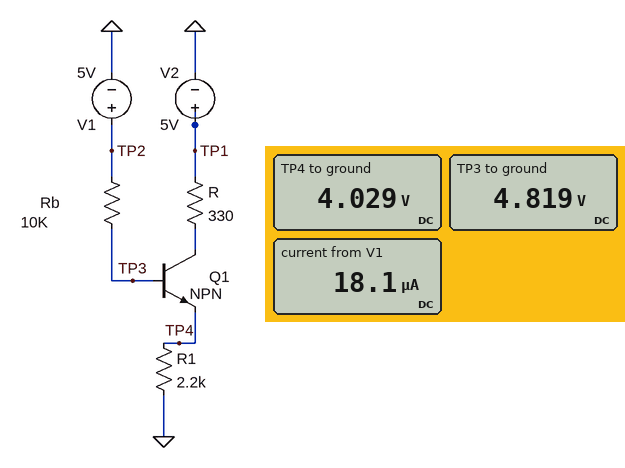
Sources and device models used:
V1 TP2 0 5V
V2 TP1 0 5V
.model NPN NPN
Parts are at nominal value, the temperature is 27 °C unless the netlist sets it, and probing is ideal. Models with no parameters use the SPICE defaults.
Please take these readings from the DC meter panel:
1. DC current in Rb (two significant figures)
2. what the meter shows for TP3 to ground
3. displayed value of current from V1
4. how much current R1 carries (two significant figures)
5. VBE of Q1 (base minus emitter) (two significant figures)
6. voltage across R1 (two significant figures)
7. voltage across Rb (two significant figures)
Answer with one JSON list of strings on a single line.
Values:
["18 µA", "4.819 V", "18.1 µA", "1.8 mA", "790 mV", "4.0 V", "180 mV"]
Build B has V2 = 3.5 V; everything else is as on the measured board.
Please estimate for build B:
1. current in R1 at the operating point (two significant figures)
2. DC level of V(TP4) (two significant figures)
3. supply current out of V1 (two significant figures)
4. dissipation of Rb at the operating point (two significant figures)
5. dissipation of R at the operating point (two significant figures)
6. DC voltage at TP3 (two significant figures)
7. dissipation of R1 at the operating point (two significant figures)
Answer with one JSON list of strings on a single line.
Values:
["1.4 mA", "3.0 V", "120 µA", "140 µW", "520 µW", "3.8 V", "4.1 mW"]
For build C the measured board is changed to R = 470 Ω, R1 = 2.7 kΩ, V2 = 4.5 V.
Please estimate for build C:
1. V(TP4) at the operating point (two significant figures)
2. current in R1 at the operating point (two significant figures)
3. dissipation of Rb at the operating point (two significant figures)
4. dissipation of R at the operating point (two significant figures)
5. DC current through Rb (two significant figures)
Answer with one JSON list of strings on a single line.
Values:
["3.8 V", "1.4 mA", "20 µW", "860 µW", "45 µA"]
